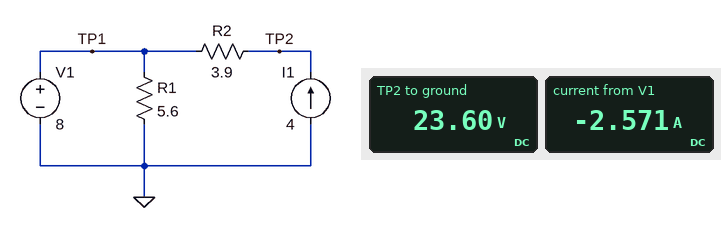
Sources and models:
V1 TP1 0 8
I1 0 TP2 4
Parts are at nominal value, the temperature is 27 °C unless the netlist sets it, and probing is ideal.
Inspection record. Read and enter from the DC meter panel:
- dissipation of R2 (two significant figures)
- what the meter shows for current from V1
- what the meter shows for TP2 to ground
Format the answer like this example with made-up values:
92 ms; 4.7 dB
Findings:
62 W; -2.571 A; 23.60 V
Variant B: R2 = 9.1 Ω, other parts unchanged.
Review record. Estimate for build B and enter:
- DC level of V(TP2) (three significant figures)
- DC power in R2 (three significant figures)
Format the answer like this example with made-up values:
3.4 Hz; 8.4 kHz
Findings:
44.4 V; 146 W
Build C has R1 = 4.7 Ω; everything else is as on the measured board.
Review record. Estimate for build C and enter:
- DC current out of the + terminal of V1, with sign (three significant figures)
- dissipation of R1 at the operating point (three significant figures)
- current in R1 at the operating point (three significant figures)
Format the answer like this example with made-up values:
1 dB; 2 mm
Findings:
-2.30 A; 13.6 W; 1.70 A
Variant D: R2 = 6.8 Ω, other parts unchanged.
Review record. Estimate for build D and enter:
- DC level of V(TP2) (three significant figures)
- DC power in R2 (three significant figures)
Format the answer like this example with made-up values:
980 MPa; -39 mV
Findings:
35.2 V; 109 W
